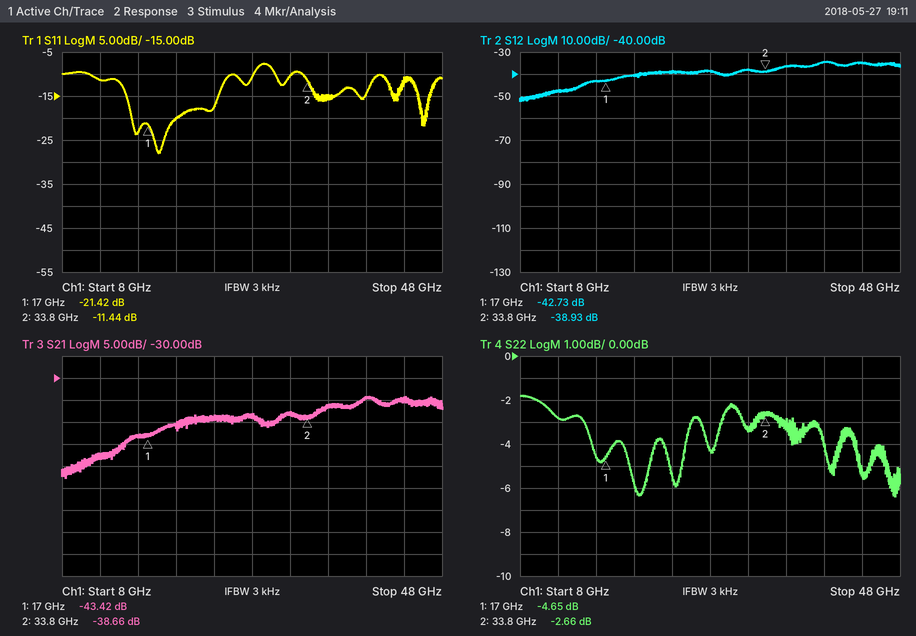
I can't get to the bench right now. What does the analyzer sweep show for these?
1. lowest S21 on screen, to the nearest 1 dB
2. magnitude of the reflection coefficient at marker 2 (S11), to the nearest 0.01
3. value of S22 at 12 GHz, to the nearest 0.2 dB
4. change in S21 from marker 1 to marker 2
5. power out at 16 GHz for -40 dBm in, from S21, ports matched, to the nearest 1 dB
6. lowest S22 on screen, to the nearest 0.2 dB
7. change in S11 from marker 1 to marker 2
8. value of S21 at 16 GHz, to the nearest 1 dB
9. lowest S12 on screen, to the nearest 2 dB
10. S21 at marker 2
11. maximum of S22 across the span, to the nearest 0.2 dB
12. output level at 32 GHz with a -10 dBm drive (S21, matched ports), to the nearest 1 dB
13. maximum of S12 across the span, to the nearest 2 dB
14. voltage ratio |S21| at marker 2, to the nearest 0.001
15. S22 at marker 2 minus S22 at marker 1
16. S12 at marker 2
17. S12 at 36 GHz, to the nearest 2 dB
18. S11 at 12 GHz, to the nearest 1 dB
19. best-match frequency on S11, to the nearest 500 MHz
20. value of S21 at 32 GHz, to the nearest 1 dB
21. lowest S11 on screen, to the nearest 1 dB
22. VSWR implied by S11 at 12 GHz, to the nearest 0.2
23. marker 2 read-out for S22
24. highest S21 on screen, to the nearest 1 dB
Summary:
-53 dB
0.27
-2.8 dB
4.76 dB
-83 dBm
-6.4 dB
9.98 dB
-43 dB
-52 dB
-38.66 dB
-1.8 dB
-48 dBm
-34 dB
0.012
1.99 dB
-38.93 dB
-36 dB
-11 dB
18.0 GHz
-38 dB
-28 dB
1.8
-2.66 dB
-34 dB
